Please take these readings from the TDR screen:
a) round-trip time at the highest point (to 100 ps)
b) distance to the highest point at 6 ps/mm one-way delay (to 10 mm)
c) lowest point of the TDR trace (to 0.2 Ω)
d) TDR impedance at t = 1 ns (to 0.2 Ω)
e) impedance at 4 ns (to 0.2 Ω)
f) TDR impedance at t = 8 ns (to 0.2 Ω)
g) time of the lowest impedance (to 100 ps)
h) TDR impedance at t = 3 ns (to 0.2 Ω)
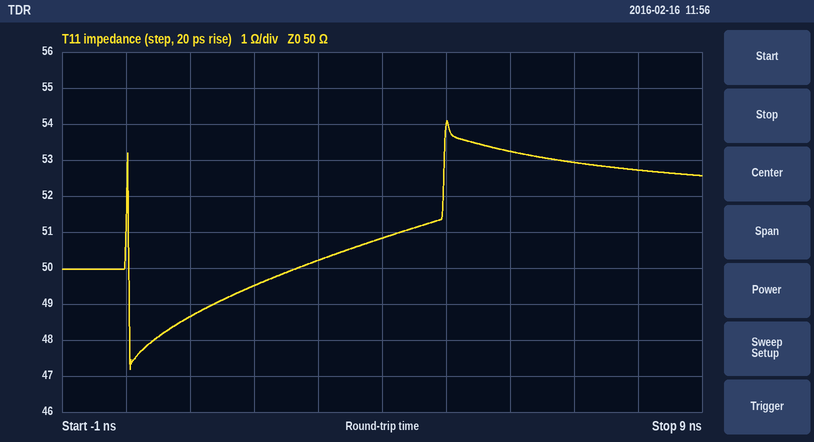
5.0 ns
420 mm
47.2 Ω
48.6 Ω
50.8 Ω
52.8 Ω
100 ps
50.2 Ω
